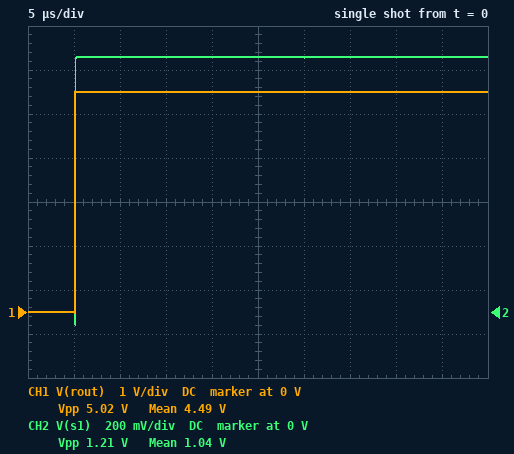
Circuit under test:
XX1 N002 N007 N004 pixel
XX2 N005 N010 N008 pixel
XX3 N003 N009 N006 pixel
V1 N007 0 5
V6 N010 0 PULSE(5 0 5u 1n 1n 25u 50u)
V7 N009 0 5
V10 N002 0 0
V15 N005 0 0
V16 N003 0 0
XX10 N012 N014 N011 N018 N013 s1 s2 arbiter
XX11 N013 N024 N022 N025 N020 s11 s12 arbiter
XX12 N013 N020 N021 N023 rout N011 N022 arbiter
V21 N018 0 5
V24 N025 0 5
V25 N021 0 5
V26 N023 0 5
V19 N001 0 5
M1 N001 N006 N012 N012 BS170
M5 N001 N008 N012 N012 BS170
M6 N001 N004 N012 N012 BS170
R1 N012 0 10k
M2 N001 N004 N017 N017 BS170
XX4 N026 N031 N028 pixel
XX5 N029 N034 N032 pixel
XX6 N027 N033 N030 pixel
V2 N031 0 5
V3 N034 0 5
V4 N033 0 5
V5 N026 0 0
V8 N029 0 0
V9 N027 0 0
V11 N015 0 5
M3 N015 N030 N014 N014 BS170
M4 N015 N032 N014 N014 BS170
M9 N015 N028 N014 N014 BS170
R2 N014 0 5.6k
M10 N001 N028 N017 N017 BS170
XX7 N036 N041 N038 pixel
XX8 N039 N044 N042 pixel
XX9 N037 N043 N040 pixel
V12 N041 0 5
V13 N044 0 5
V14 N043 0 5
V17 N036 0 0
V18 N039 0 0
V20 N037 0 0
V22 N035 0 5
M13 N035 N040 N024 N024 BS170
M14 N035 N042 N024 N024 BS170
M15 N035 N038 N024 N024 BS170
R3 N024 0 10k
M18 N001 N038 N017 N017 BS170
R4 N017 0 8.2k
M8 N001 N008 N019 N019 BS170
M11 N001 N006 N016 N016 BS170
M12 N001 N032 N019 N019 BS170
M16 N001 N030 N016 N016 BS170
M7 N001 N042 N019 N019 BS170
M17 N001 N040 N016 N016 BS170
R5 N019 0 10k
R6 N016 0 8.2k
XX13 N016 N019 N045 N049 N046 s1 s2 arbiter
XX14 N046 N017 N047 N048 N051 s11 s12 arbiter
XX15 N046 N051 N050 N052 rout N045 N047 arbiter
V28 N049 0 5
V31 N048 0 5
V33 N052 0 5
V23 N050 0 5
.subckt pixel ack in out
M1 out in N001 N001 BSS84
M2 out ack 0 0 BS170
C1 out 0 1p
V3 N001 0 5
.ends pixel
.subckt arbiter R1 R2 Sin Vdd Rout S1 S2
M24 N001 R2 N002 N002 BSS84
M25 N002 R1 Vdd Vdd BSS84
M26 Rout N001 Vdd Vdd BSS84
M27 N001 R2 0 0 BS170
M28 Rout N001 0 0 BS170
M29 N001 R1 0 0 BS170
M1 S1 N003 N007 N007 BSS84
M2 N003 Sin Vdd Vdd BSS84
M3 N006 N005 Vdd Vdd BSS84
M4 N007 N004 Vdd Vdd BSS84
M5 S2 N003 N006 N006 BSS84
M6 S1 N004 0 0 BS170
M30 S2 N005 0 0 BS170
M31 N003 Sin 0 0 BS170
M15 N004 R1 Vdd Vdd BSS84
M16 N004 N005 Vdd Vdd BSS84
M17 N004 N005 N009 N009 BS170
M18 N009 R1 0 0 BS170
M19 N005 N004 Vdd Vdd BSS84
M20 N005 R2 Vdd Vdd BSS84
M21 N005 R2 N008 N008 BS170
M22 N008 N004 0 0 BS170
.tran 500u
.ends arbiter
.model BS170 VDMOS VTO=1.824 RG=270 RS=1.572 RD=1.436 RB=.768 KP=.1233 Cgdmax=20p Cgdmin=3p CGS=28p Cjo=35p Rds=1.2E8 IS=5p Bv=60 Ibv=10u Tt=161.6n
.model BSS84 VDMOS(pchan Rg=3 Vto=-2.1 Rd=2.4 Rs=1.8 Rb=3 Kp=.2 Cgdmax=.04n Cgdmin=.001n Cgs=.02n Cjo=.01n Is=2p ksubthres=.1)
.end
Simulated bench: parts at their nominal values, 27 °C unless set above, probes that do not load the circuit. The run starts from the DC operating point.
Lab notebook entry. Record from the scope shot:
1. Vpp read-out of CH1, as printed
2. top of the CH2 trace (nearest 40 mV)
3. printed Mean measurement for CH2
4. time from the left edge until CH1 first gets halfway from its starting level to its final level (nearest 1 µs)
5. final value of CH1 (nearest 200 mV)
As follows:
5.02 V
1.16 V
1.04 V
5 µs
5.0 V
